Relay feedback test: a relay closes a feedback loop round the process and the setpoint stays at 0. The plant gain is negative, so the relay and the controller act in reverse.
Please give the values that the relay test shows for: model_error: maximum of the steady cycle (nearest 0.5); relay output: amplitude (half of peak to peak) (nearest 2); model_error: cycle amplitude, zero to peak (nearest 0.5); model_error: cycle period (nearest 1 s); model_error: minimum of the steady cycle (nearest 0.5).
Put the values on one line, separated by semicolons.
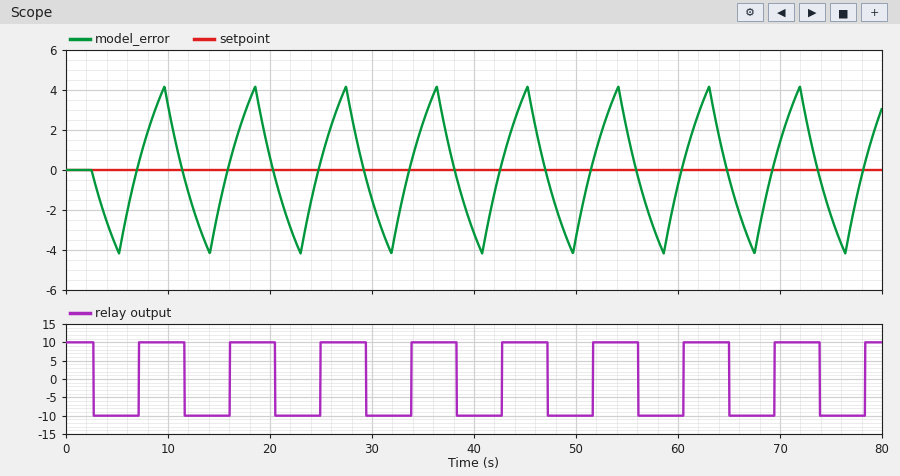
4.0; 10; 4.0; 9 s; -4.0
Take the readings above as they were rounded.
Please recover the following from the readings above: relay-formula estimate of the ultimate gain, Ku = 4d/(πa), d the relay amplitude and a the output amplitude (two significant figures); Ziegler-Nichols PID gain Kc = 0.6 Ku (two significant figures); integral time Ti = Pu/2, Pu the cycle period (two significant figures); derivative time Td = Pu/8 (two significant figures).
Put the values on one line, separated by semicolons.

3.2; 1.9; 4.5 s; 1.1 s
